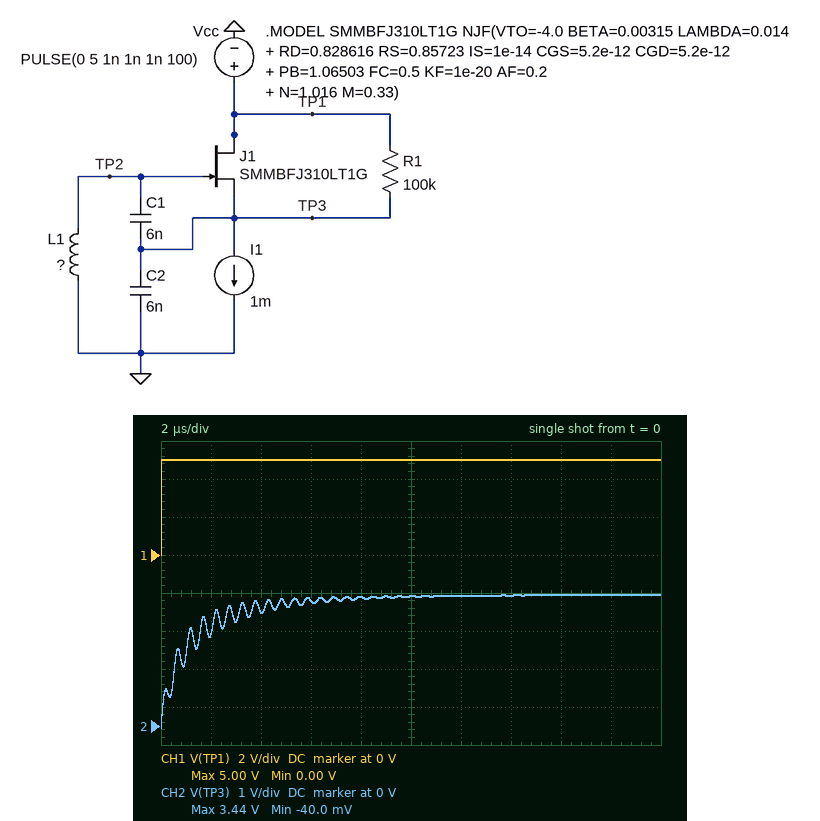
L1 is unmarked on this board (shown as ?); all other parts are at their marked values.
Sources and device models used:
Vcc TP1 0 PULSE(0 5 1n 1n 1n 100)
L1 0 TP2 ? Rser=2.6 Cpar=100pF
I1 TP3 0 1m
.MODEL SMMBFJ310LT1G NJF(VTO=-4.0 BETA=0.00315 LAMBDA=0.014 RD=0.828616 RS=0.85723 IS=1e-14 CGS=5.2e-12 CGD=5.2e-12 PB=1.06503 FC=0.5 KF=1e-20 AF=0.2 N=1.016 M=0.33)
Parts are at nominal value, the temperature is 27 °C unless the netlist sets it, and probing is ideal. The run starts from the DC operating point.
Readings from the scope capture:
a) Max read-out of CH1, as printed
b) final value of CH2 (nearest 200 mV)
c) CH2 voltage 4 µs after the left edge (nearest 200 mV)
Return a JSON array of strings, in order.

["5.00 V", "3.4 V", "3.0 V"]
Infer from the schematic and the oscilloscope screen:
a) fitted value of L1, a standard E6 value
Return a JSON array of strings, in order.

["2.2 µH"]
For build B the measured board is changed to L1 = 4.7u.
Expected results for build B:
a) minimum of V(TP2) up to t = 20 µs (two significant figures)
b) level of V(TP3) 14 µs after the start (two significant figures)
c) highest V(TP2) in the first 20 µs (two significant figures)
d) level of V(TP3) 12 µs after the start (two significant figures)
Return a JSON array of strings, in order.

["-1.6 V", "3.5 V", "1.6 V", "3.3 V"]
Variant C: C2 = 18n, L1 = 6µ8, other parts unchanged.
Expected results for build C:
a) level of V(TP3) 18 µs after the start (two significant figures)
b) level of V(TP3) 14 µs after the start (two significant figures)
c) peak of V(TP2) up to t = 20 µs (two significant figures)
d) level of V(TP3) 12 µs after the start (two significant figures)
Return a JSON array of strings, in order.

["3.5 V", "3.3 V", "700 mV", "3.2 V"]
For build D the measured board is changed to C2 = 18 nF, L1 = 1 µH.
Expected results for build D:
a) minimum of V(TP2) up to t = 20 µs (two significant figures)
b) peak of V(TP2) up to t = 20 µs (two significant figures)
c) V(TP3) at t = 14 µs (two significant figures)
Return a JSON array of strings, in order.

["-140 mV", "200 mV", "3.3 V"]
